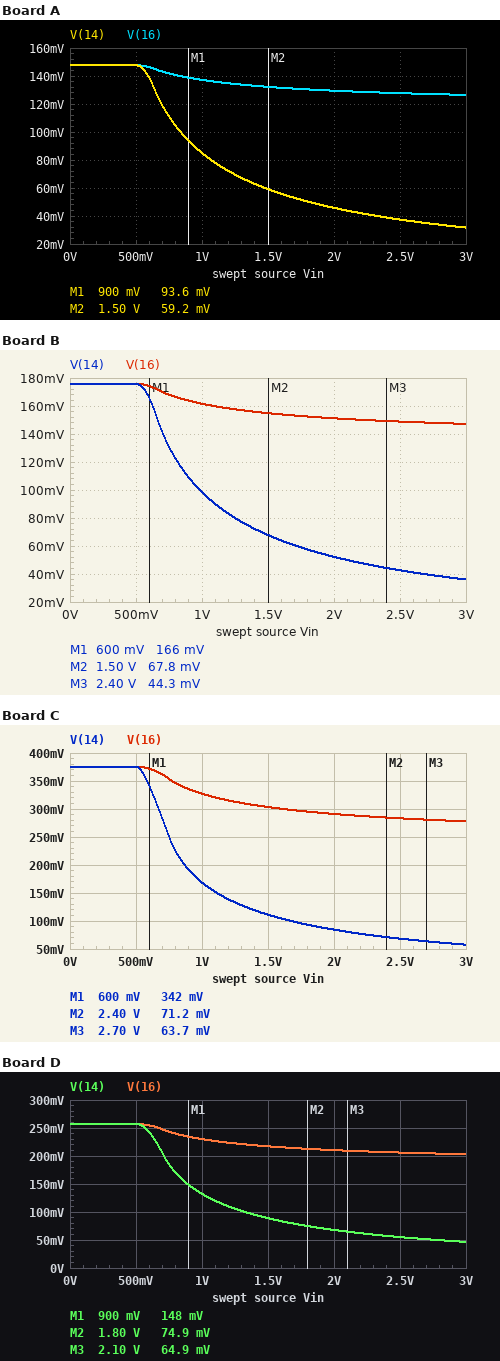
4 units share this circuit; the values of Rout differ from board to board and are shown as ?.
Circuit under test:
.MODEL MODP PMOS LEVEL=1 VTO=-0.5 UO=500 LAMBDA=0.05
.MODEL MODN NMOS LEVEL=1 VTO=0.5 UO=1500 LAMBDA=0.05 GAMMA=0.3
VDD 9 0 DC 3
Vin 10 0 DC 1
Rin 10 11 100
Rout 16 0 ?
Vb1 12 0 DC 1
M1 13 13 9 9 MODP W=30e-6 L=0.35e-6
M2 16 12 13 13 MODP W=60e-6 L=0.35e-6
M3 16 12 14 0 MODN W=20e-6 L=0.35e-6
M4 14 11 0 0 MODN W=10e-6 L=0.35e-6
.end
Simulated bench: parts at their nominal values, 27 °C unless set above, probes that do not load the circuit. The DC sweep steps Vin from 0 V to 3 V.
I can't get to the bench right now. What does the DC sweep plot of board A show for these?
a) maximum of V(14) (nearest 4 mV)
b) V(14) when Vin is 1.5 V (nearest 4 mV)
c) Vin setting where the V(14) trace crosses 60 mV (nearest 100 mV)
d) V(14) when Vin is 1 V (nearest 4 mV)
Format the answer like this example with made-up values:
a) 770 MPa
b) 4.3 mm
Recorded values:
a) 148 mV
b) 60 mV
c) 1.5 V
d) 84 mV
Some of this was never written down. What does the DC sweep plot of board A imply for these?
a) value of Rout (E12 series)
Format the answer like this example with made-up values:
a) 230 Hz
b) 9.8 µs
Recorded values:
a) 470 Ω
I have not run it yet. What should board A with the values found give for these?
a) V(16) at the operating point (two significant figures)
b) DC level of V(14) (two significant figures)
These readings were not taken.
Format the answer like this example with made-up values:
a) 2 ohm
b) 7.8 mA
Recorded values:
a) 140 mV
b) 85 mV
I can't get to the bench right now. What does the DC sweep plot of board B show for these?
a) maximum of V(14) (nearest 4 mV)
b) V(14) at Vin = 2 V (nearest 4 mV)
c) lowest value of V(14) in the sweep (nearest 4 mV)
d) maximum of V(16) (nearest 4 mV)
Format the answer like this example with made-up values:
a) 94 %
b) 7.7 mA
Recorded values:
a) 176 mV
b) 52 mV
c) 36 mV
d) 176 mV
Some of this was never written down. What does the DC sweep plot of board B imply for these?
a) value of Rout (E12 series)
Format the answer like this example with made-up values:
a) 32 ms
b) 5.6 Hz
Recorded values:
a) 560 Ω
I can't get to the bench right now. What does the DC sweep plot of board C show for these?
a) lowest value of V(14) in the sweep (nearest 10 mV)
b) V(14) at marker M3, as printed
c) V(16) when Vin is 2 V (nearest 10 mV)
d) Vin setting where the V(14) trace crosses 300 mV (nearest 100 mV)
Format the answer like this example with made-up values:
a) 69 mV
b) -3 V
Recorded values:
a) 60 mV
b) 63.7 mV
c) 290 mV
d) 700 mV
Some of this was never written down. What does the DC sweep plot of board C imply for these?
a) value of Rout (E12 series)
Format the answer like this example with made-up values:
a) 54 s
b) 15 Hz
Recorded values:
a) 1.2 kΩ
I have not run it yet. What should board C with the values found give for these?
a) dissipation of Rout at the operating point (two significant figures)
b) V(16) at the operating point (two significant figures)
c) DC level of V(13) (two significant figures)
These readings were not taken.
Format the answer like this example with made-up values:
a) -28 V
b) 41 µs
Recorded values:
a) 89 µW
b) 330 mV
c) 1.9 V
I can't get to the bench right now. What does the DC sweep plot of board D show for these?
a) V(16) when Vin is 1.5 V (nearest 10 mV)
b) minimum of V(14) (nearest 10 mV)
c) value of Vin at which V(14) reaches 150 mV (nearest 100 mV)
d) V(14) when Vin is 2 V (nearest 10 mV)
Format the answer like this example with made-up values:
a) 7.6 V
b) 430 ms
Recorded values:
a) 220 mV
b) 50 mV
c) 900 mV
d) 70 mV
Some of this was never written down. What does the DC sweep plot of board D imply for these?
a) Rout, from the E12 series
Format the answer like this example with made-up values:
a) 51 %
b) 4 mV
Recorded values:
a) 820 Ω
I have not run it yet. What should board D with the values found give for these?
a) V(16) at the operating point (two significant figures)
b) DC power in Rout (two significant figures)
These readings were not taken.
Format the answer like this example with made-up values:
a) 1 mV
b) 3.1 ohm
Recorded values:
a) 230 mV
b) 65 µW
